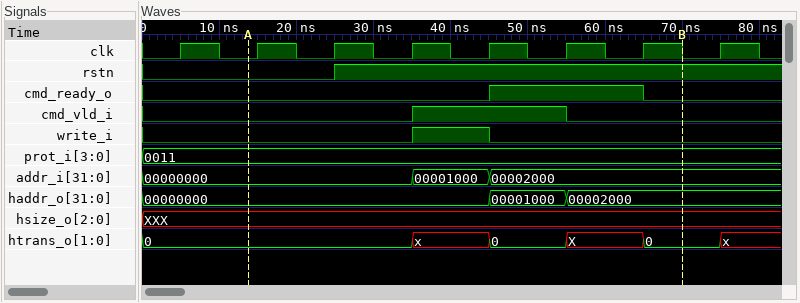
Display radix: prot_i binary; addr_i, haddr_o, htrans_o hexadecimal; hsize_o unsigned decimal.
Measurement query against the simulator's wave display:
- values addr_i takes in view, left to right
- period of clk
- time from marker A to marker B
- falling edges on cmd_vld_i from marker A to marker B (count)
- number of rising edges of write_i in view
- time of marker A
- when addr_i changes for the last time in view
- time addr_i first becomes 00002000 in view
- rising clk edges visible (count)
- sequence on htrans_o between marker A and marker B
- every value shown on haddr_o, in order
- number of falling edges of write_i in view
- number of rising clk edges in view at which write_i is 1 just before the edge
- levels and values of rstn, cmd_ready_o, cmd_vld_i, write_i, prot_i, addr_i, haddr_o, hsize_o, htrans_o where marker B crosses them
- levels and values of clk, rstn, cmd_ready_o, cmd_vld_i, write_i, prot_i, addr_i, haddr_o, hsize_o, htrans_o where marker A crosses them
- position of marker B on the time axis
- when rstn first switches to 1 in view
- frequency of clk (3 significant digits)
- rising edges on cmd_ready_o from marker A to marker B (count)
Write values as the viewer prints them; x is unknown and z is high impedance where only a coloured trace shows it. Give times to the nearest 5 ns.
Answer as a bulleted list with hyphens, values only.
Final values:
- 00000000, 00001000, 00002000
- 10 ns
- 55 ns
- 1
- 1
- 15 ns
- 45 ns
- 45 ns
- 8
- 0, x, 0, X, 0
- 00000000, 00001000, 00002000
- 1
- 1
- rstn=1, cmd_ready_o=0, cmd_vld_i=0, write_i=0, prot_i=0011, addr_i=00002000, haddr_o=00002000, hsize_o=XXX, htrans_o=0
- clk=0, rstn=0, cmd_ready_o=0, cmd_vld_i=0, write_i=0, prot_i=0011, addr_i=00000000, haddr_o=00000000, hsize_o=XXX, htrans_o=0
- 70 ns
- 25 ns
- 100 MHz
- 1
